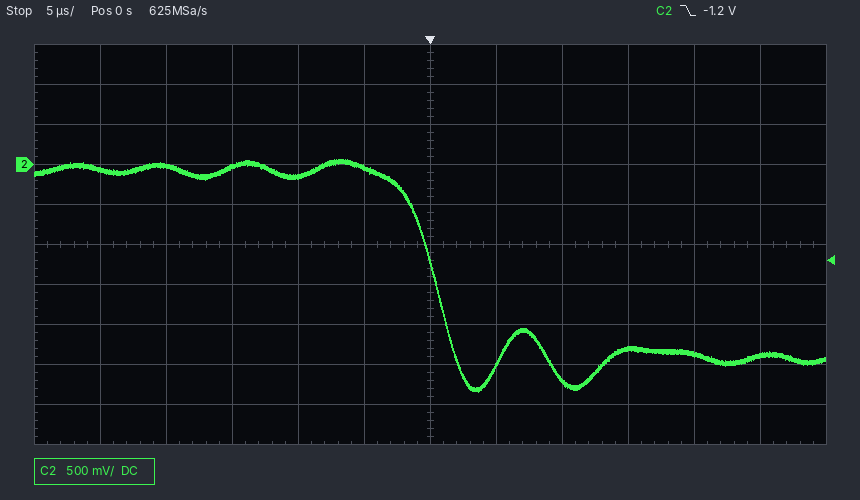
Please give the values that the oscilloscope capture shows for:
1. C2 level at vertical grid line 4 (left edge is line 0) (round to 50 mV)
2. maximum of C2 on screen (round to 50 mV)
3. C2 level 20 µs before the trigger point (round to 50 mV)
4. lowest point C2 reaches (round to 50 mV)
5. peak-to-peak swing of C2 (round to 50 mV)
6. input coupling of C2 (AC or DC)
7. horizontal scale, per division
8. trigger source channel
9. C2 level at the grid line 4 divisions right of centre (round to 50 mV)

-150 mV
50 mV
0 mV
-2.85 V
2.90 V
DC
5 µs
C2
-2.35 V
